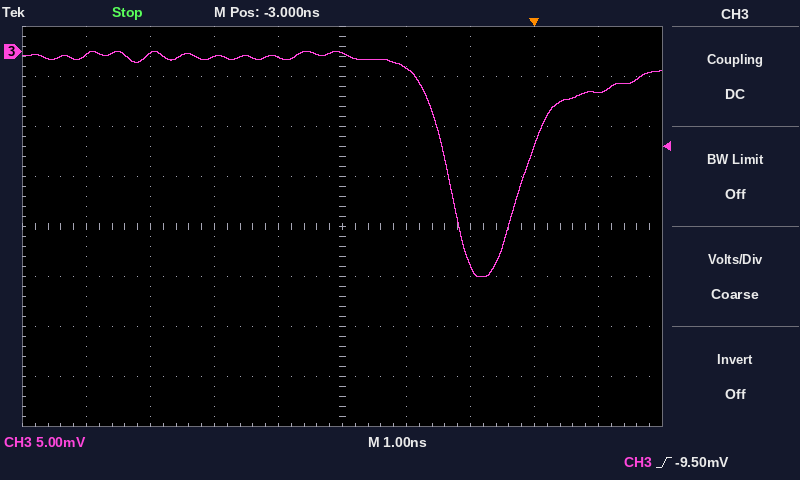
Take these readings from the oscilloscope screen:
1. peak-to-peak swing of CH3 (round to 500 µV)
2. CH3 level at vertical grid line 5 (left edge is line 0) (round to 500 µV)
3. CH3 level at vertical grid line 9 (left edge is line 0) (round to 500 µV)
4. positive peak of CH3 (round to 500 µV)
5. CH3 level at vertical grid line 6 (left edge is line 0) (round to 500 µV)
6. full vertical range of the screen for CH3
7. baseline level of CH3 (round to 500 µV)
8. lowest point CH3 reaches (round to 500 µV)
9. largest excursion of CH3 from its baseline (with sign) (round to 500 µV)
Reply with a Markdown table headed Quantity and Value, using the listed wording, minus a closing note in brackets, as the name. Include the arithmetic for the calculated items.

| Quantity | Value |
|---|---|
| peak-to-peak swing of CH3 | 0.0 mV − (-22.5 mV) = 22.5 mV |
| CH3 level at vertical grid line 5 (left edge is line 0) | 0.0 mV |
| CH3 level at vertical grid line 9 (left edge is line 0) | -4.0 mV |
| positive peak of CH3 | 0.0 mV |
| CH3 level at vertical grid line 6 (left edge is line 0) | -1.5 mV |
| full vertical range of the screen for CH3 | 40 mV |
| baseline level of CH3 | -500 µV |
| lowest point CH3 reaches | -22.5 mV |
| largest excursion of CH3 from its baseline (with sign) | -22.5 mV − (-500 µV) = -22.0 mV |
